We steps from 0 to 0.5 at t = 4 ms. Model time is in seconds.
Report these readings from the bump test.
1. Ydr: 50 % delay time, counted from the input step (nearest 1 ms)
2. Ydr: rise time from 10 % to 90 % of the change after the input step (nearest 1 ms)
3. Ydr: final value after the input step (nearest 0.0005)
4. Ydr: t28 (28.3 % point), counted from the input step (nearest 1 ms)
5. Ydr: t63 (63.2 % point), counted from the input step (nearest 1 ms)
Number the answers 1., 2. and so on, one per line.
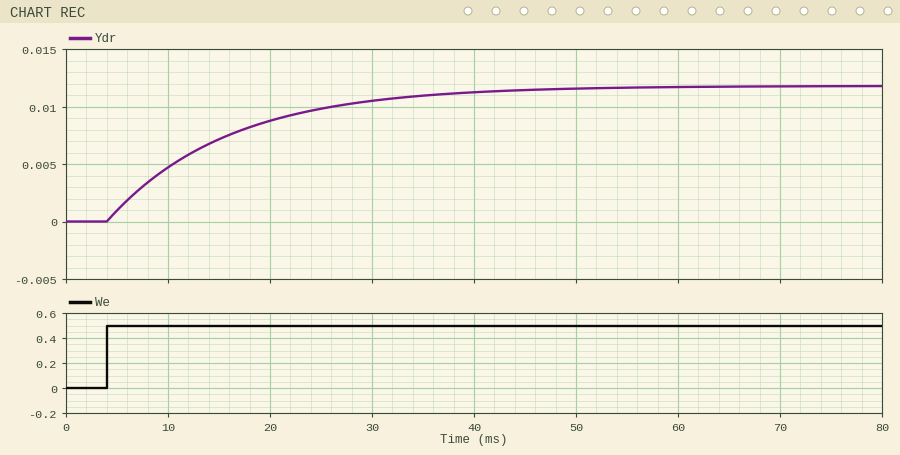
1. 8 ms
2. 26 ms
3. 0.0120
4. 4 ms
5. 12 ms
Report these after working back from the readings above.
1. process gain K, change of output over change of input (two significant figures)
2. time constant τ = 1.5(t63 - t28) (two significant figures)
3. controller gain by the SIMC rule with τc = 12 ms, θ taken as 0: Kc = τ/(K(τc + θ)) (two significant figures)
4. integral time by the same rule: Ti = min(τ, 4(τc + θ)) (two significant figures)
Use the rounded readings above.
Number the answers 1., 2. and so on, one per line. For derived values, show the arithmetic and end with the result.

1. (0.012 - 0) / 0.5 = 0.024
2. 1.5 × (12 - 4) = 12 ms
3. 12 / (0.024 × (12 + 0)) = 42
4. min(12, 4 × (12 + 0)) = 12 ms
